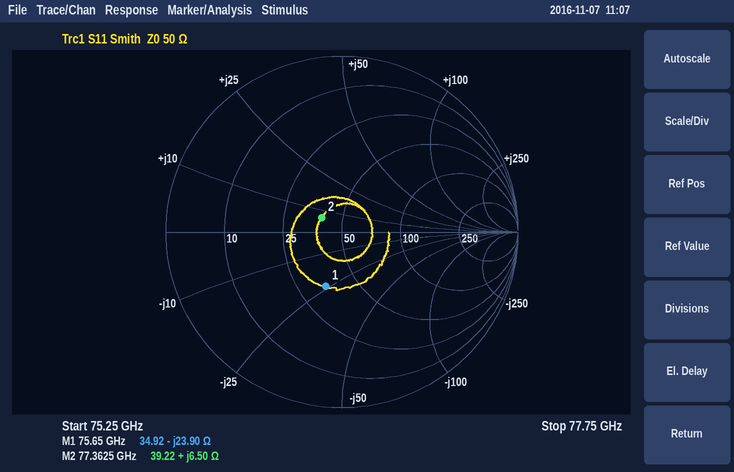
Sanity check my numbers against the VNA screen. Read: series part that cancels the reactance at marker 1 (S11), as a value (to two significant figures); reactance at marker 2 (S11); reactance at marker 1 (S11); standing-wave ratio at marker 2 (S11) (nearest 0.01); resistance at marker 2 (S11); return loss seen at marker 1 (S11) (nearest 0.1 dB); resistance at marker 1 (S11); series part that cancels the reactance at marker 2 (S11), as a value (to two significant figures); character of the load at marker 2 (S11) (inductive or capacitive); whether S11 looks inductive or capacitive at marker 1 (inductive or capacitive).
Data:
50 pH
+6.50 Ω
-23.90 Ω
1.33
39.22 Ω
9.9 dB
34.92 Ω
320 fF
inductive
capacitive
